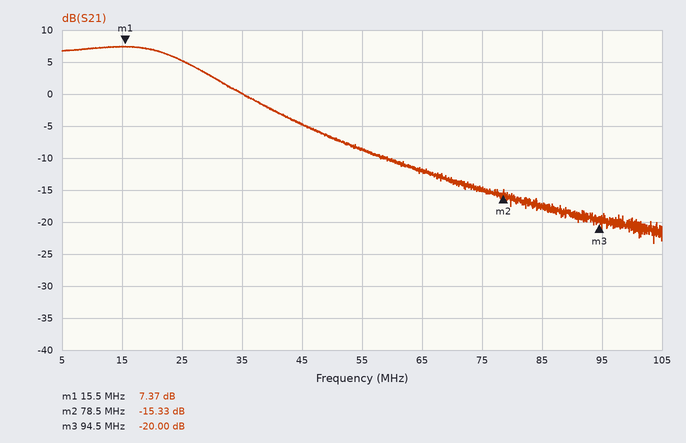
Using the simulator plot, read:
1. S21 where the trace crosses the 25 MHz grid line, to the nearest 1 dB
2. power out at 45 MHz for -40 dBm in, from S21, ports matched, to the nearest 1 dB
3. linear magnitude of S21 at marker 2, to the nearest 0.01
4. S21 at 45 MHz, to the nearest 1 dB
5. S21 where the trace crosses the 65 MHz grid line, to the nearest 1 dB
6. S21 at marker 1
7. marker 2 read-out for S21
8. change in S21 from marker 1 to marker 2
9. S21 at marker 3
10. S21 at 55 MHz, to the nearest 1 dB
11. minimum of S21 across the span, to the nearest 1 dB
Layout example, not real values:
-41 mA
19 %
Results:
5 dB
-45 dBm
0.17
-5 dB
-12 dB
7.37 dB
-15.33 dB
-22.70 dB
-20.00 dB
-9 dB
-23 dB
